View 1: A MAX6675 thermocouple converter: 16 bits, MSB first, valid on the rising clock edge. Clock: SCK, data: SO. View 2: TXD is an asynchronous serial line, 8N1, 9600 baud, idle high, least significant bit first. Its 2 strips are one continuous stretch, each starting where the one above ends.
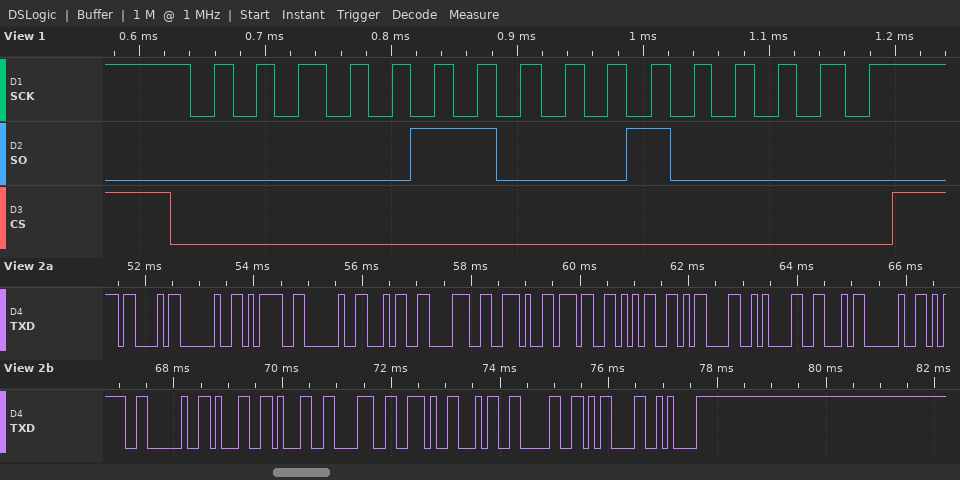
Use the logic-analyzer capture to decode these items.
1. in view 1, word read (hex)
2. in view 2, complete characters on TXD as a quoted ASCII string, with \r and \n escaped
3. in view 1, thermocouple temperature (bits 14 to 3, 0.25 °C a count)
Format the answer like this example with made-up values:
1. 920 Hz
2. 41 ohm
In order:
1. 0x0620
2. "C = 48.75\r\nF = 118.40\r\n"
3. 49.00 °C
